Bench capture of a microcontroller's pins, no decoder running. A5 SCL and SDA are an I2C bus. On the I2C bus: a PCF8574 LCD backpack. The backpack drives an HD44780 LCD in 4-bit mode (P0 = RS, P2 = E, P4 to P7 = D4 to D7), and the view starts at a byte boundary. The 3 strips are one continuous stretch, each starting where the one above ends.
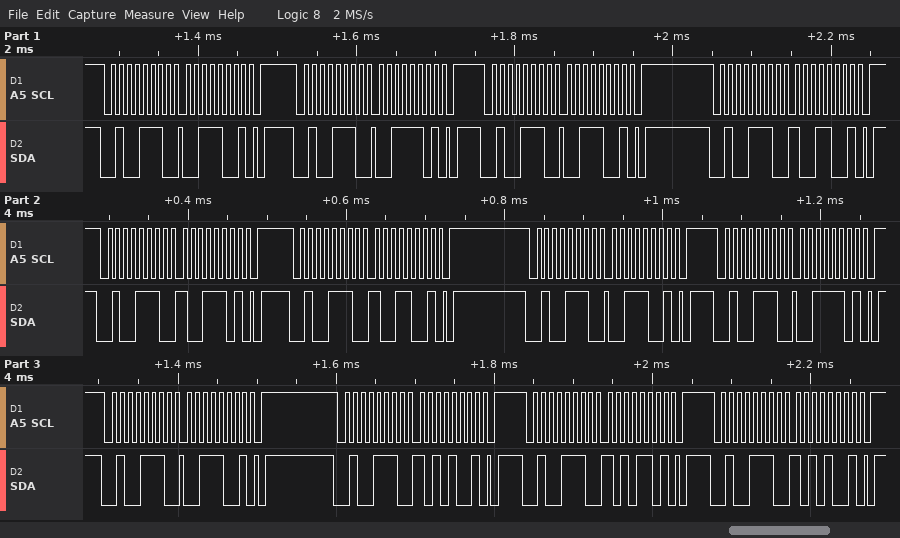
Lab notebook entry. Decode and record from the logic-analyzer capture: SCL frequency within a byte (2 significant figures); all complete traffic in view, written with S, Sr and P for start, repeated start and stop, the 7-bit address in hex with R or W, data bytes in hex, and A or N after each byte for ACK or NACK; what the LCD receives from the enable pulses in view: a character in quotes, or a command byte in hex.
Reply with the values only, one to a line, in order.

100 kHz
S 27W A 39 A P S 27W A 3D A P S 27W A 39 A P S 27W A 99 A P S 27W A 9D A P S 27W A 99 A P S 27W A 39 A P S 27W A 3D A P S 27W A 39 A P S 27W A A9 A P S 27W A AD A P S 27W A A9 A P
'9' ':'
